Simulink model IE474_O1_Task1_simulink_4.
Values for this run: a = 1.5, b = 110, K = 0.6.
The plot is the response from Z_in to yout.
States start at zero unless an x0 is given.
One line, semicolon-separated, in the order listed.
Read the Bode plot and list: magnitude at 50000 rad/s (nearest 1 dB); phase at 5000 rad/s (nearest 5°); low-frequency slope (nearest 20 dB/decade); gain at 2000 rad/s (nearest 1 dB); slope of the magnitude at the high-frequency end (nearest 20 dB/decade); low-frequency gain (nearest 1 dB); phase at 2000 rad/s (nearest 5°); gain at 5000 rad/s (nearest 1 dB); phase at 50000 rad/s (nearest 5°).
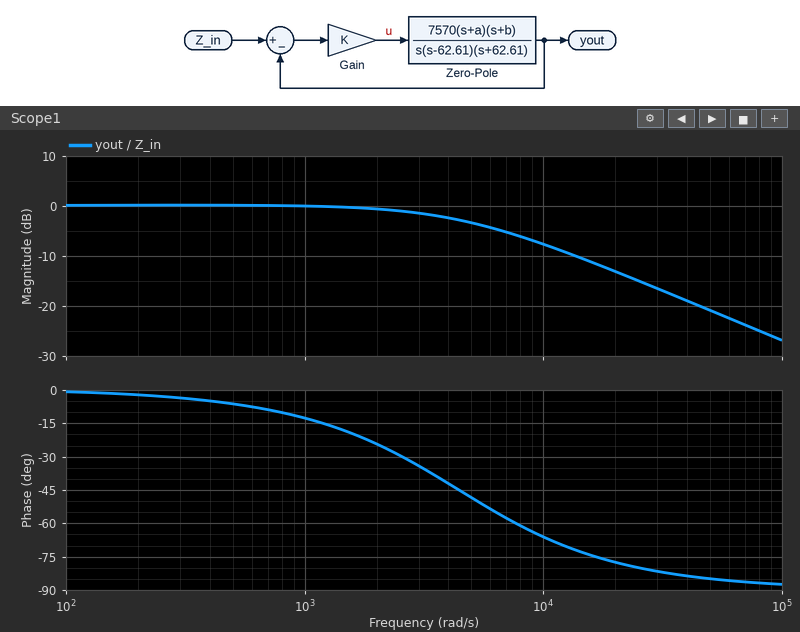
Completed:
-21 dB; -50°; 0 dB/decade; -1 dB; -20 dB/decade; 0 dB; -25°; -3 dB; -85°
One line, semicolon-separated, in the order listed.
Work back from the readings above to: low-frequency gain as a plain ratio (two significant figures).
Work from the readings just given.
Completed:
1.0
